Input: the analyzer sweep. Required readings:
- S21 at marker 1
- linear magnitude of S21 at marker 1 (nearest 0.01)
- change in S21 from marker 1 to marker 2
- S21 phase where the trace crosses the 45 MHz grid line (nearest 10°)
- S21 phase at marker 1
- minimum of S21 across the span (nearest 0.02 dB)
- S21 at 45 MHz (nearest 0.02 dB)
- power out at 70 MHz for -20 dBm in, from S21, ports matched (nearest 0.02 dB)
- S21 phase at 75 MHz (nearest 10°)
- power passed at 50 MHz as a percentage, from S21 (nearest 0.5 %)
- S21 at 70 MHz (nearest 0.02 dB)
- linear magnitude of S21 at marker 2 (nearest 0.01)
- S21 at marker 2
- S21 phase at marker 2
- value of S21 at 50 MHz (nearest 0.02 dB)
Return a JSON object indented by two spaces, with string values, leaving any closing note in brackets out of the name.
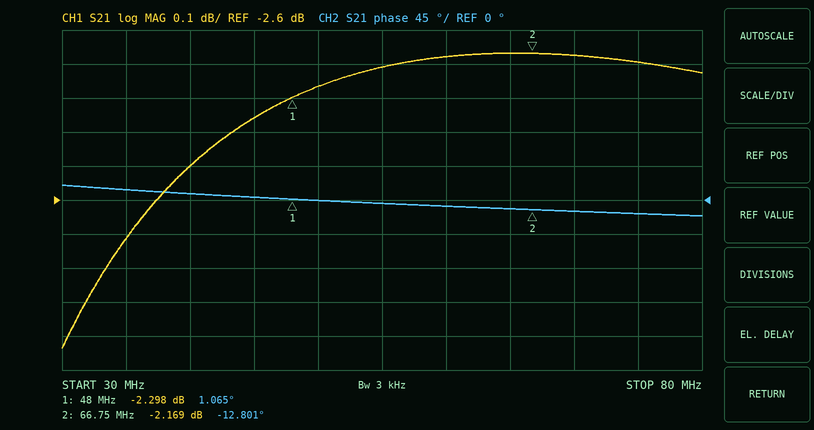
{
  "S21 at marker 1": "-2.298 dB",
  "linear magnitude of S21 at marker 1": "0.77",
  "change in S21 from marker 1 to marker 2": "0.129 dB",
  "S21 phase where the trace crosses the 45 MHz grid line": "0°",
  "S21 phase at marker 1": "1.065°",
  "minimum of S21 across the span": "-3.04 dB",
  "S21 at 45 MHz": "-2.36 dB",
  "power out at 70 MHz for -20 dBm in, from S21, ports matched": "-22.18 dBm",
  "S21 phase at 75 MHz": "-20°",
  "power passed at 50 MHz as a percentage, from S21": "59.5 %",
  "S21 at 70 MHz": "-2.18 dB",
  "linear magnitude of S21 at marker 2": "0.78",
  "S21 at marker 2": "-2.169 dB",
  "S21 phase at marker 2": "-12.801°",
  "value of S21 at 50 MHz": "-2.26 dB"
}
